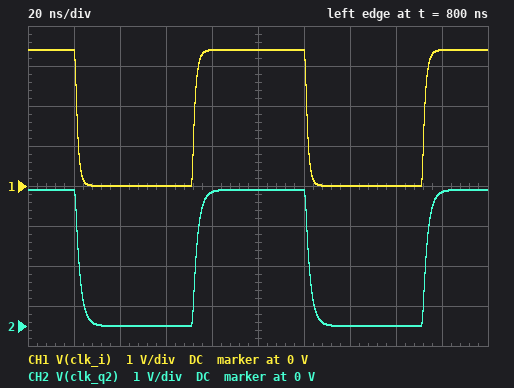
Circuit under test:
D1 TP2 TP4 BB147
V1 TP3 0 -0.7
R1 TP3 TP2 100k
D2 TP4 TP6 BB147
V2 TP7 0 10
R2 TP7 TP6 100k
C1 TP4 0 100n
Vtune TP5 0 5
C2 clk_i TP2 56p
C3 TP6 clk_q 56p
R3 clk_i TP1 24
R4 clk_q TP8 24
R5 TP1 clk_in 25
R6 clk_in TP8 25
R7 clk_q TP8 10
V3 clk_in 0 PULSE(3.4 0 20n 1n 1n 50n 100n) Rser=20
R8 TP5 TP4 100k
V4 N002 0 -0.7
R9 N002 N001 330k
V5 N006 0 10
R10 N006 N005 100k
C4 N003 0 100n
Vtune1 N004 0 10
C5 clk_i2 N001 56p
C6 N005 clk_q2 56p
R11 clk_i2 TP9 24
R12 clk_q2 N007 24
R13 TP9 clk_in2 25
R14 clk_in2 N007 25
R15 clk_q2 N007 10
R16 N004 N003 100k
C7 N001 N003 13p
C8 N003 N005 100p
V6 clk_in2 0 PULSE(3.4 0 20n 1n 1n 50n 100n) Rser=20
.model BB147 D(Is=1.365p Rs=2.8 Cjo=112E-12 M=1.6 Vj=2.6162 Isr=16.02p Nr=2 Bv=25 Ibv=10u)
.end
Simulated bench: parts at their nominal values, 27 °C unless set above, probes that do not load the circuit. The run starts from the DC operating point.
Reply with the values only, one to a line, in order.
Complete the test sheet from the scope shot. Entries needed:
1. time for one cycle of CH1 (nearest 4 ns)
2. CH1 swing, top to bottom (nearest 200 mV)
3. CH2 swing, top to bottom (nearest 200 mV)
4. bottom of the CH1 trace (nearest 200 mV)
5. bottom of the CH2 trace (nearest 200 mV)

100 ns
3.4 V
3.4 V
0 V
0 V
